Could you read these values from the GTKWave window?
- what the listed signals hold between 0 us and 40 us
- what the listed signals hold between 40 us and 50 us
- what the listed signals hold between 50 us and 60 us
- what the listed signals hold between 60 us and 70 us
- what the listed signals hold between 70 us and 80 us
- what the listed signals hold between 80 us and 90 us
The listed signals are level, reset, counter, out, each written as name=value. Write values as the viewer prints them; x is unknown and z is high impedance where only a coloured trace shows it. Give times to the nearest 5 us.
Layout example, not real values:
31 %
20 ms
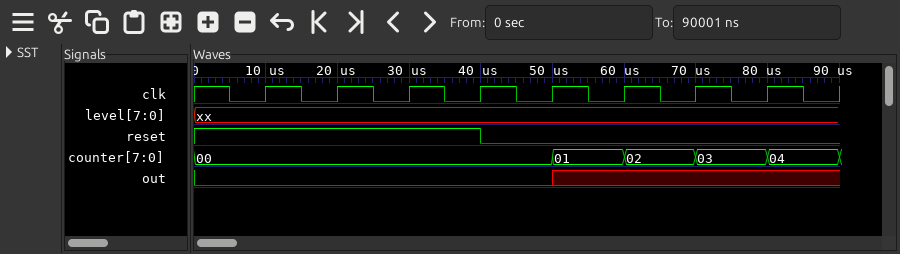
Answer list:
level=xx, reset=1, counter=00, out=0
level=xx, reset=0, counter=00, out=0
level=xx, reset=0, counter=01, out=x
level=xx, reset=0, counter=02, out=x
level=xx, reset=0, counter=03, out=x
level=xx, reset=0, counter=04, out=x
